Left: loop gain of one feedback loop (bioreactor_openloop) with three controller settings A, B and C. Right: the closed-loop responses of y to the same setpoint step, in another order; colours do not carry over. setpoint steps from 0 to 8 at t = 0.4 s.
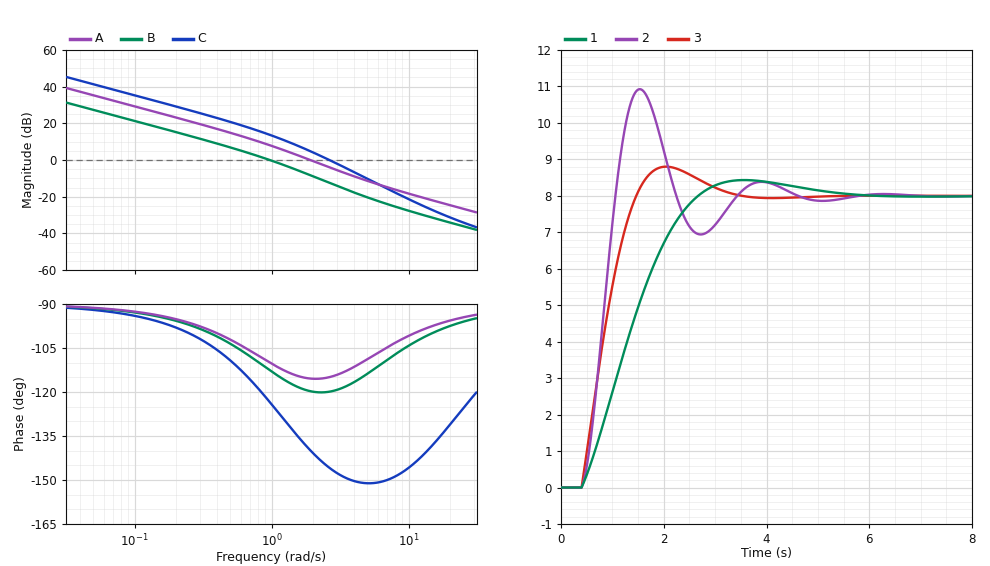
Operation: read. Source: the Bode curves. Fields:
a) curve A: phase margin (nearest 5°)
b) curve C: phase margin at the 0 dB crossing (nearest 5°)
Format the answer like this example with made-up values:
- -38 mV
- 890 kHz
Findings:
- 65°
- 35°
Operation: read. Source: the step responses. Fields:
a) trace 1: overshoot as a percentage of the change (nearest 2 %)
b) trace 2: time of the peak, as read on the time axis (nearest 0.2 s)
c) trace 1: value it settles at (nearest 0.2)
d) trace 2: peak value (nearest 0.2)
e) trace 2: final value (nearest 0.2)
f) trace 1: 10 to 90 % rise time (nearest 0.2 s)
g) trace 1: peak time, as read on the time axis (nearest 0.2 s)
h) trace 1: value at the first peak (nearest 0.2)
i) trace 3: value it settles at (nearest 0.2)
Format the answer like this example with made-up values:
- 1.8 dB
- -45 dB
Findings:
- 6 %
- 1.6 s
- 8.0
- 11.0
- 8.0
- 1.6 s
- 3.6 s
- 8.4
- 8.0
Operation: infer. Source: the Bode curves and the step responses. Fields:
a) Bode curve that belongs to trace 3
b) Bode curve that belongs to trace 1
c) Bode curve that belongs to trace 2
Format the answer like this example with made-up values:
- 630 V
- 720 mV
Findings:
- A
- B
- C
